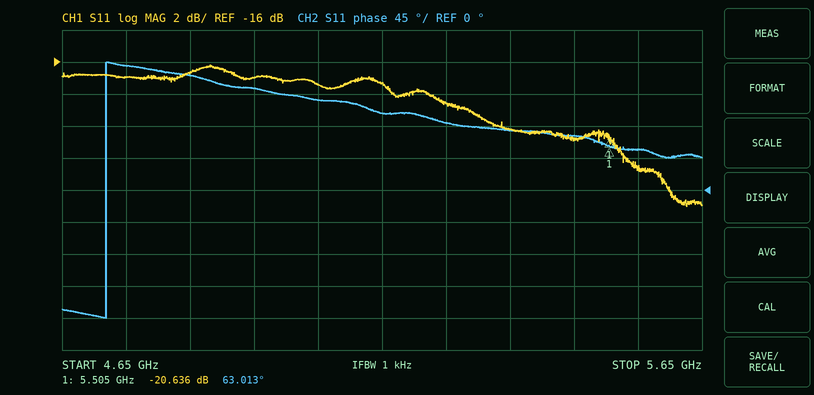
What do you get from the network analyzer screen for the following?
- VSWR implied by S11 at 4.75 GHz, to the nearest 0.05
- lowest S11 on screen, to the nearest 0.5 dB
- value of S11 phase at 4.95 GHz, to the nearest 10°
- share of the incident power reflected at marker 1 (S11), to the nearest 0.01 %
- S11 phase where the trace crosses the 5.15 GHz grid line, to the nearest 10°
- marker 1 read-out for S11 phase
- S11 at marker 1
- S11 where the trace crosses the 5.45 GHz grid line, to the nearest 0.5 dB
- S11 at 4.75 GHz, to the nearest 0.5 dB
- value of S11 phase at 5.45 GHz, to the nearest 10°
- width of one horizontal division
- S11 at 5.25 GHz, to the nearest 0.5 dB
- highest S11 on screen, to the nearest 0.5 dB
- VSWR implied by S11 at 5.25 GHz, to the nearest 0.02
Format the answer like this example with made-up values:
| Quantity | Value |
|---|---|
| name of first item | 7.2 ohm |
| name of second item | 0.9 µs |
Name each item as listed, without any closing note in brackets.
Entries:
| Quantity | Value |
|---|---|
| VSWR implied by S11 at 4.75 GHz, to the nearest 0.05 | 1.35 |
| lowest S11 on screen, to the nearest 0.5 dB | -25.0 dB |
| value of S11 phase at 4.95 GHz, to the nearest 10° | 140° |
| share of the incident power reflected at marker 1 (S11), to the nearest 0.01 % | 0.86 % |
| S11 phase where the trace crosses the 5.15 GHz grid line, to the nearest 10° | 110° |
| marker 1 read-out for S11 phase | 63.013° |
| S11 at marker 1 | -20.636 dB |
| S11 where the trace crosses the 5.45 GHz grid line, to the nearest 0.5 dB | -21.0 dB |
| S11 at 4.75 GHz, to the nearest 0.5 dB | -17.0 dB |
| value of S11 phase at 5.45 GHz, to the nearest 10° | 80° |
| width of one horizontal division | 100 MHz |
| S11 at 5.25 GHz, to the nearest 0.5 dB | -18.5 dB |
| highest S11 on screen, to the nearest 0.5 dB | -16.0 dB |
| VSWR implied by S11 at 5.25 GHz, to the nearest 0.02 | 1.26 |
